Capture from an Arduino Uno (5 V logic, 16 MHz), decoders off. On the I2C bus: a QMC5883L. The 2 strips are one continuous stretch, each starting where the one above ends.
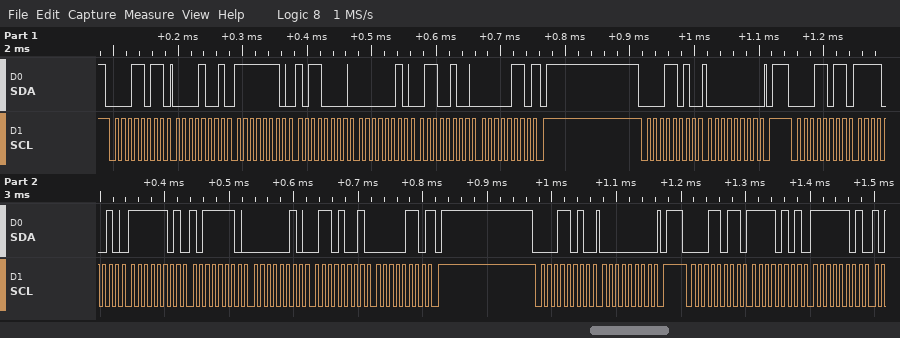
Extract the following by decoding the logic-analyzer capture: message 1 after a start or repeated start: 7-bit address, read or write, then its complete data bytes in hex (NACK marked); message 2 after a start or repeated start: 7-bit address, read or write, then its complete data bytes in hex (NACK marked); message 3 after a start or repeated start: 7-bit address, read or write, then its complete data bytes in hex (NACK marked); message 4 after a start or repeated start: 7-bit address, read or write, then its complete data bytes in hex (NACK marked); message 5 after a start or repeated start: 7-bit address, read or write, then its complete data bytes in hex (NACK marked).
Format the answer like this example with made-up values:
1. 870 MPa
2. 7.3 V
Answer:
1. 0x0D read: 09 FE B0 02 64 06 NACK
2. 0x0D write: 00
3. 0x0D read: F2 FD BE 02 69 06 NACK
4. 0x0D write: 00
5. 0x0D read: F5 FD
